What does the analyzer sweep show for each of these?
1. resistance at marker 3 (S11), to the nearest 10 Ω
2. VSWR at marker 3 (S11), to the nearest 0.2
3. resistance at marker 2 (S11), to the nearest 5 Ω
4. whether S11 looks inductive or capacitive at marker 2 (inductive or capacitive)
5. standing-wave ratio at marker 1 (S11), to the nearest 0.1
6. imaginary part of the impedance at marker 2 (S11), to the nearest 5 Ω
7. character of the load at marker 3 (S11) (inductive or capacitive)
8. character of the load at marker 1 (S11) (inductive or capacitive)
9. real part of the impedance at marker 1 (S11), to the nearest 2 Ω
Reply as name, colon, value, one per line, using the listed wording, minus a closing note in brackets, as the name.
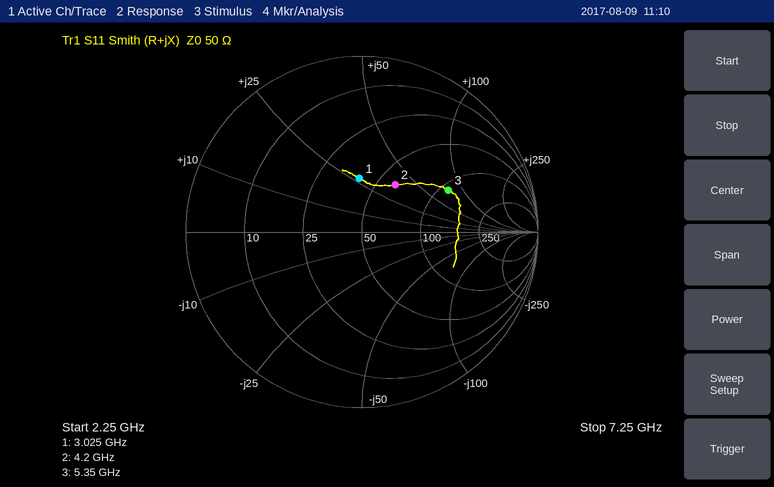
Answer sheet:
resistance at marker 3 (S11), to the nearest 10 Ω: 110 Ω
VSWR at marker 3 (S11), to the nearest 0.2: 3.4
resistance at marker 2 (S11), to the nearest 5 Ω: 60 Ω
whether S11 looks inductive or capacitive at marker 2: inductive
standing-wave ratio at marker 1 (S11), to the nearest 0.1: 1.9
imaginary part of the impedance at marker 2 (S11), to the nearest 5 Ω: +35 Ω
character of the load at marker 3 (S11): inductive
character of the load at marker 1 (S11): inductive
real part of the impedance at marker 1 (S11), to the nearest 2 Ω: 40 Ω
